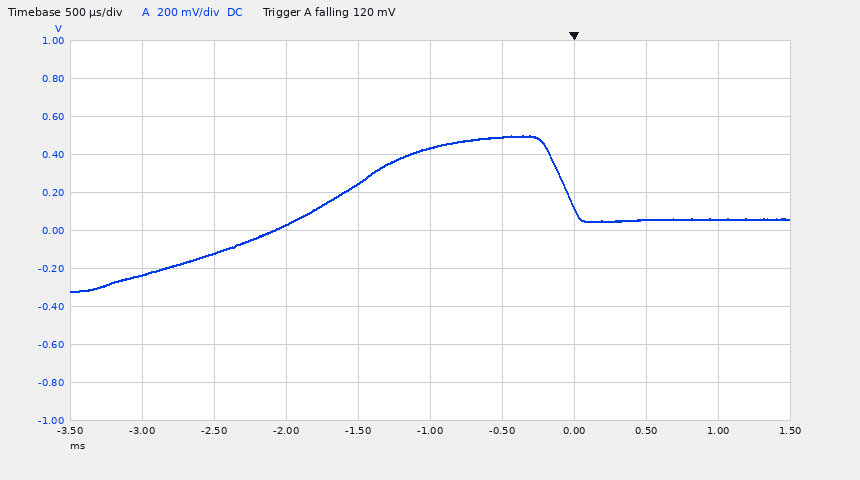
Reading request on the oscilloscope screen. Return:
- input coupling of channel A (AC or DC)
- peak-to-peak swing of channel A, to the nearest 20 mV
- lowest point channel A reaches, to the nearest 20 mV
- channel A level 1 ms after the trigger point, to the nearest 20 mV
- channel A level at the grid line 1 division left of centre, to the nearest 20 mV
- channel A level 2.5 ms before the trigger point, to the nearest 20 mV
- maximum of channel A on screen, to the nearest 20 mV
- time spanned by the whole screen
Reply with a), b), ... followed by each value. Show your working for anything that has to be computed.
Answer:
a) DC
b) 500 mV − (-320 mV) = 820 mV
c) -320 mV
d) 60 mV
e) 240 mV
f) -120 mV
g) 500 mV
h) 5 ms
